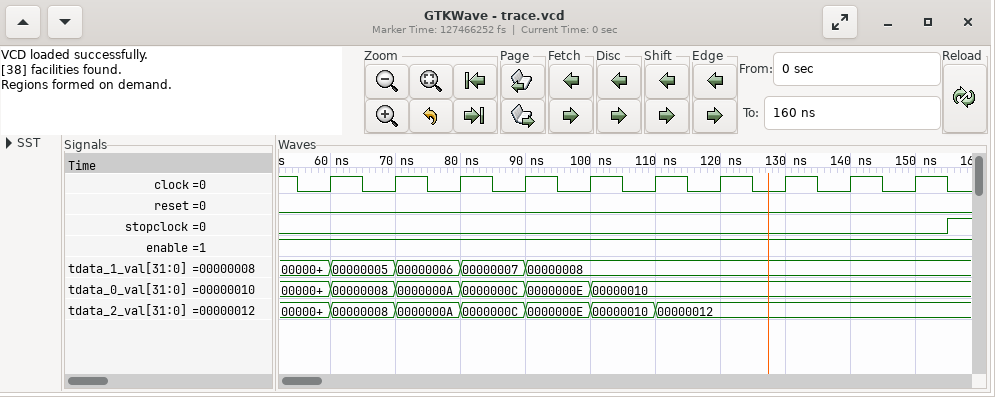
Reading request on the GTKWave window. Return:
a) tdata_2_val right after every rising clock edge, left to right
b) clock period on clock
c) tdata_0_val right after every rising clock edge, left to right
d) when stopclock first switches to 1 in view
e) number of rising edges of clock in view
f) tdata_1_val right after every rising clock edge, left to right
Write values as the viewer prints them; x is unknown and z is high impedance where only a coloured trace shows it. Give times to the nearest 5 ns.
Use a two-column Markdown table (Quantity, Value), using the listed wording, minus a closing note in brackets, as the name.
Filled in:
| Quantity | Value |
|---|---|
| tdata_2_val right after every rising clock edge, left to right | 00000008, 0000000A, 0000000C, 0000000E, 00000010, 00000012, 00000012, 00000012, 00000012, 00000012 |
| clock period on clock | 10 ns |
| tdata_0_val right after every rising clock edge, left to right | 00000008, 0000000A, 0000000C, 0000000E, 00000010, 00000010, 00000010, 00000010, 00000010, 00000010 |
| when stopclock first switches to 1 in view | 155 ns |
| number of rising edges of clock in view | 10 |
| tdata_1_val right after every rising clock edge, left to right | 00000005, 00000006, 00000007, 00000008, 00000008, 00000008, 00000008, 00000008, 00000008, 00000008 |
